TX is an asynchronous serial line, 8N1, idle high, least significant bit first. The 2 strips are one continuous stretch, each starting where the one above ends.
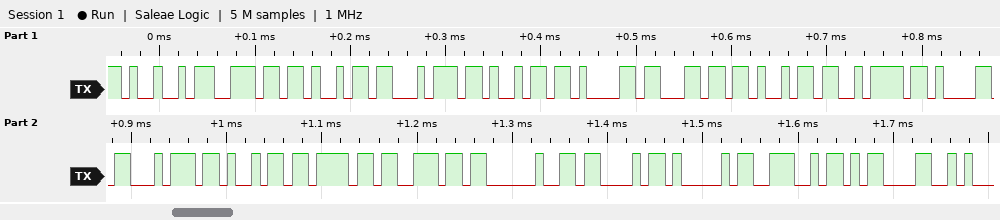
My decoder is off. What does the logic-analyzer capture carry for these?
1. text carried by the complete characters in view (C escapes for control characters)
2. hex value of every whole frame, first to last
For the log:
"Initialization CAN\r"
0x49 0x6E 0x69 0x74 0x69 0x61 0x6C 0x69 0x7A 0x61 0x74 0x69 0x6F 0x6E 0x20 0x43 0x41 0x4E 0x0D
